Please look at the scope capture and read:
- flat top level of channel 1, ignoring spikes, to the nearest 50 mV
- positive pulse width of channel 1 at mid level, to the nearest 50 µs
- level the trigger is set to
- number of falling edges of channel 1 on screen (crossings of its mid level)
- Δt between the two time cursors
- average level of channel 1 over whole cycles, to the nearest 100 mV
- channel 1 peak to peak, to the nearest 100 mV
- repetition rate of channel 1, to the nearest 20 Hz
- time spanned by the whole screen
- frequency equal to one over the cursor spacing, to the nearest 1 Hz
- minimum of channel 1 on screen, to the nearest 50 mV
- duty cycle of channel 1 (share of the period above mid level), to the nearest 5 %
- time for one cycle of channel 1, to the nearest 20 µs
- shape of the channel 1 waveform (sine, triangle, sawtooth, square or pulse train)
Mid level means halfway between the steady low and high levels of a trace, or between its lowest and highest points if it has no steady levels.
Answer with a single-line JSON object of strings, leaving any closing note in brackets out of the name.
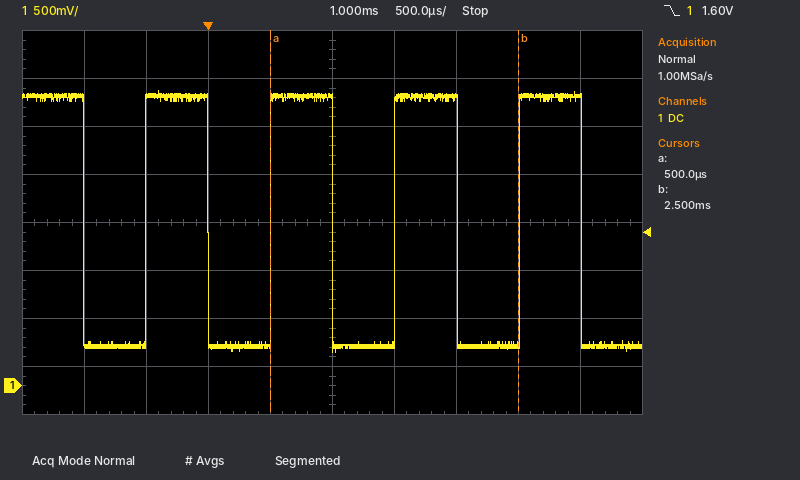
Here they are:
{"flat top level of channel 1, ignoring spikes, to the nearest 50 mV": "3.00 V", "positive pulse width of channel 1 at mid level, to the nearest 50 µs": "500 µs", "level the trigger is set to": "1.60 V", "number of falling edges of channel 1 on screen": "5", "Δt between the two time cursors": "2.00 ms", "average level of channel 1 over whole cycles, to the nearest 100 mV": "1.7 V", "channel 1 peak to peak, to the nearest 100 mV": "2.70 V", "repetition rate of channel 1, to the nearest 20 Hz": "1.00 kHz", "time spanned by the whole screen": "5 ms", "frequency equal to one over the cursor spacing, to the nearest 1 Hz": "500 Hz", "minimum of channel 1 on screen, to the nearest 50 mV": "350 mV", "duty cycle of channel 1 (share of the period above mid level), to the nearest 5 %": "50 %", "time for one cycle of channel 1, to the nearest 20 µs": "1.00 ms", "shape of the channel 1 waveform": "square"}
